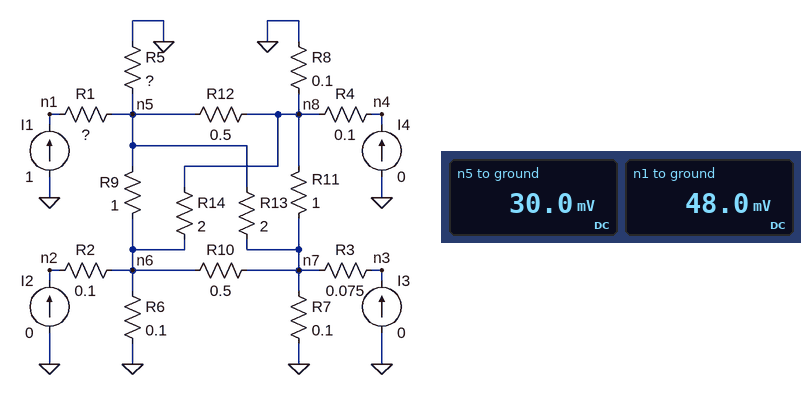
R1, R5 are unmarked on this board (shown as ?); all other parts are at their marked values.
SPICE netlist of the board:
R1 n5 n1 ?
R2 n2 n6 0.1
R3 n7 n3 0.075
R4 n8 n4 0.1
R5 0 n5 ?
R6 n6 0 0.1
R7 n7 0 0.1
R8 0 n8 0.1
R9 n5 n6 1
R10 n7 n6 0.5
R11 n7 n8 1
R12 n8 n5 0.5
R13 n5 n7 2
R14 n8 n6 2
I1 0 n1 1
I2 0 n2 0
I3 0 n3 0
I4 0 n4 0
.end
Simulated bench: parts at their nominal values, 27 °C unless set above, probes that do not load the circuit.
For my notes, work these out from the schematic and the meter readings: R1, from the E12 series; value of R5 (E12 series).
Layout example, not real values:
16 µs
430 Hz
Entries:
0.018 Ω
0.033 Ω
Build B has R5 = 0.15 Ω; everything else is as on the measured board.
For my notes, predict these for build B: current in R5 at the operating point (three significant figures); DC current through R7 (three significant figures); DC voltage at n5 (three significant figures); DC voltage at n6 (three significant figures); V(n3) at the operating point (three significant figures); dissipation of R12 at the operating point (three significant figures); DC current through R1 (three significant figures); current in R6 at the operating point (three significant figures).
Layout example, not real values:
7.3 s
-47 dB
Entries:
685 mA
63.5 mA
103 mV
9.14 mV
6.35 mV
15.0 mW
1.00 A
91.4 mA
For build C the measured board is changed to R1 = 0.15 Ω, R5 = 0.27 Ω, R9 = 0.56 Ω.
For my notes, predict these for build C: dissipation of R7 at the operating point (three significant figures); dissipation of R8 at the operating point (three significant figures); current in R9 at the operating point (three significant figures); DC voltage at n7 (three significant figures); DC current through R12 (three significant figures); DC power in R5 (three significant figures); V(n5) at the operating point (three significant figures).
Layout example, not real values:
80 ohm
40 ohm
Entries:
887 µW
4.60 mW
208 mA
9.42 mV
228 mA
67.9 mW
135 mV
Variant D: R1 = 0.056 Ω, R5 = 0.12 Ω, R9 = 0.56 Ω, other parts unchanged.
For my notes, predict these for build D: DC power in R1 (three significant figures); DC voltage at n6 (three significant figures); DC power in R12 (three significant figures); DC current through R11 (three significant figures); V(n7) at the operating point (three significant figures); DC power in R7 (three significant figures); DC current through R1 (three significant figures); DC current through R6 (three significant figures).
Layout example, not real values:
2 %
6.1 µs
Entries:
56.0 mW
11.7 mV
9.81 mW
7.40 mA
5.79 mV
335 µW
1.00 A
117 mA
